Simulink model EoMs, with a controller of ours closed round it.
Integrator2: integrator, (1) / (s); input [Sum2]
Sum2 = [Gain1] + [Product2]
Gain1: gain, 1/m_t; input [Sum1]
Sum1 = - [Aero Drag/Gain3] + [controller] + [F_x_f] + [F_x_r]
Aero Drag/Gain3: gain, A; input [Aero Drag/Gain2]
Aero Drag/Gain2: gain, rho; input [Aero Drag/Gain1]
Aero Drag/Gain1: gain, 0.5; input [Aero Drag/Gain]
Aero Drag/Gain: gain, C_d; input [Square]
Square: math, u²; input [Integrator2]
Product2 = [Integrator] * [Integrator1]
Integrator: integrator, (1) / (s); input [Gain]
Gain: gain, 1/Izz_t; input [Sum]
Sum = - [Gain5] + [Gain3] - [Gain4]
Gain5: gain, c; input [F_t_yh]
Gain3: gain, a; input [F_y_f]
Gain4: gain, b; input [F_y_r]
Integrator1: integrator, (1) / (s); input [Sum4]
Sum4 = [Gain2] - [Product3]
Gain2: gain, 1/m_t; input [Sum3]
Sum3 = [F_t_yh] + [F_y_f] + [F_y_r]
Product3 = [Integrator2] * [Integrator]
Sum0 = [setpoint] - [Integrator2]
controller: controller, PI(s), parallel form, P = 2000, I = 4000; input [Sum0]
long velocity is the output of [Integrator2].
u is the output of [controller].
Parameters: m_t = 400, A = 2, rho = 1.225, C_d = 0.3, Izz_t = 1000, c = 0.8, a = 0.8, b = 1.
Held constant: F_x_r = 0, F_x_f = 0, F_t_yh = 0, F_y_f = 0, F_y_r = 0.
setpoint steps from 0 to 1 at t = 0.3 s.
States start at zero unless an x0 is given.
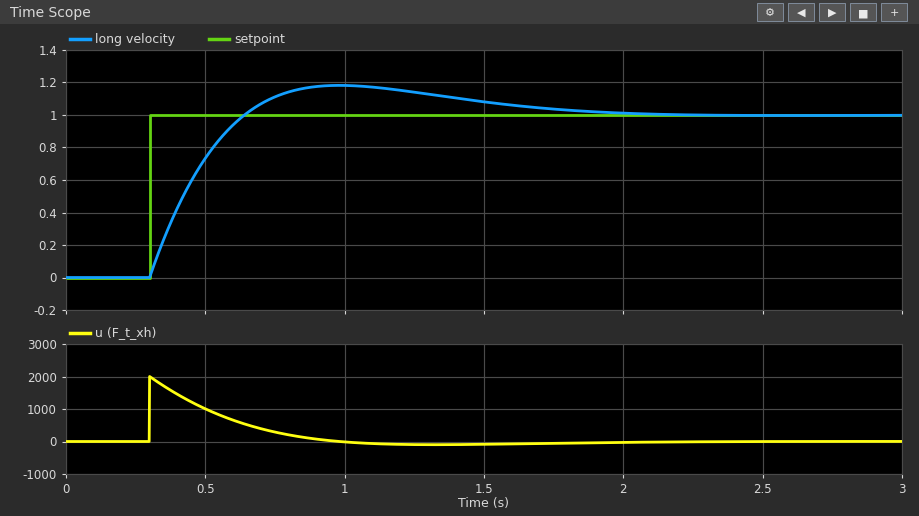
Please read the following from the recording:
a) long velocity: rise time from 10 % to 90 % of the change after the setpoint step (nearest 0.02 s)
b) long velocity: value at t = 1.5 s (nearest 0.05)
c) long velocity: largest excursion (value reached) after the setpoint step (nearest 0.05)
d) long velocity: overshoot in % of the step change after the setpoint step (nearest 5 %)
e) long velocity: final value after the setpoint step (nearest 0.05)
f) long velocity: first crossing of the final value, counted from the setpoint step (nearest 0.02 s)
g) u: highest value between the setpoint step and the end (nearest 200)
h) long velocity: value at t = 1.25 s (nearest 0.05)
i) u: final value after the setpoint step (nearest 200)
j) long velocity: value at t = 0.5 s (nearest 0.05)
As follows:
0.26 s
1.10
1.20
20 %
1.00
0.34 s
2000
1.15
0
0.75
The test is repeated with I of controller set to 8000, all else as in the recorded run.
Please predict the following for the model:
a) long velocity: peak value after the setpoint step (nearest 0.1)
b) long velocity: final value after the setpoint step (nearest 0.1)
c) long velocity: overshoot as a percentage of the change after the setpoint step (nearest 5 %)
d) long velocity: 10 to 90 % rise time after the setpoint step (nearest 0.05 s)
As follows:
1.3
1.0
25 %
0.20 s
